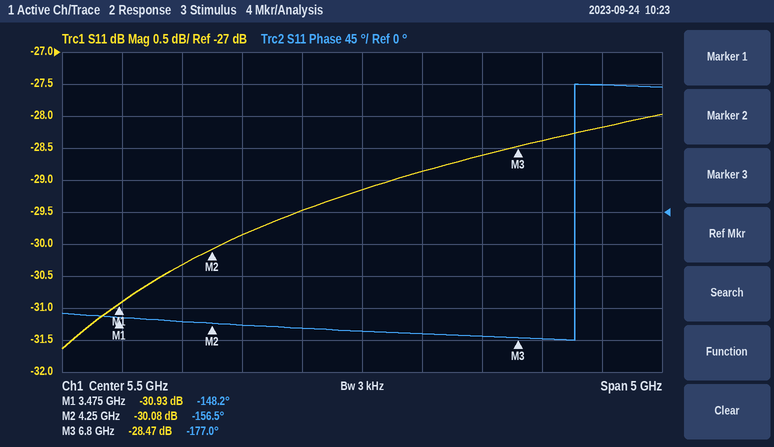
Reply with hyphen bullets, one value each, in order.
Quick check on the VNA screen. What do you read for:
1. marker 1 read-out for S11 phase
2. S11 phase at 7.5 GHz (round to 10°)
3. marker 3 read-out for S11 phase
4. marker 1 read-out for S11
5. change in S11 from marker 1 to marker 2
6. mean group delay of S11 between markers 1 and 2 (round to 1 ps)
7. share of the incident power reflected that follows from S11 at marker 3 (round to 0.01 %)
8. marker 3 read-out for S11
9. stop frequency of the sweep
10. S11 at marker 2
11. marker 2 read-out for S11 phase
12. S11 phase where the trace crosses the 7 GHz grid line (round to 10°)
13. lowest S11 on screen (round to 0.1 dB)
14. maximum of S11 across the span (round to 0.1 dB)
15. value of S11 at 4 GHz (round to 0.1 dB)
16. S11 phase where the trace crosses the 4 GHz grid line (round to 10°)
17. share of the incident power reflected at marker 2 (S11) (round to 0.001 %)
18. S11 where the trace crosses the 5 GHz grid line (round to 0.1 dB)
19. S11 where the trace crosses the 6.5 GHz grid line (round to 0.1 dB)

- -148.2°
- 180°
- -177.0°
- -30.93 dB
- 0.85 dB
- 30 ps
- 0.14 %
- -28.47 dB
- 8 GHz
- -30.08 dB
- -156.5°
- -180°
- -31.6 dB
- -28.0 dB
- -30.3 dB
- -150°
- 0.098 %
- -29.5 dB
- -28.6 dB
